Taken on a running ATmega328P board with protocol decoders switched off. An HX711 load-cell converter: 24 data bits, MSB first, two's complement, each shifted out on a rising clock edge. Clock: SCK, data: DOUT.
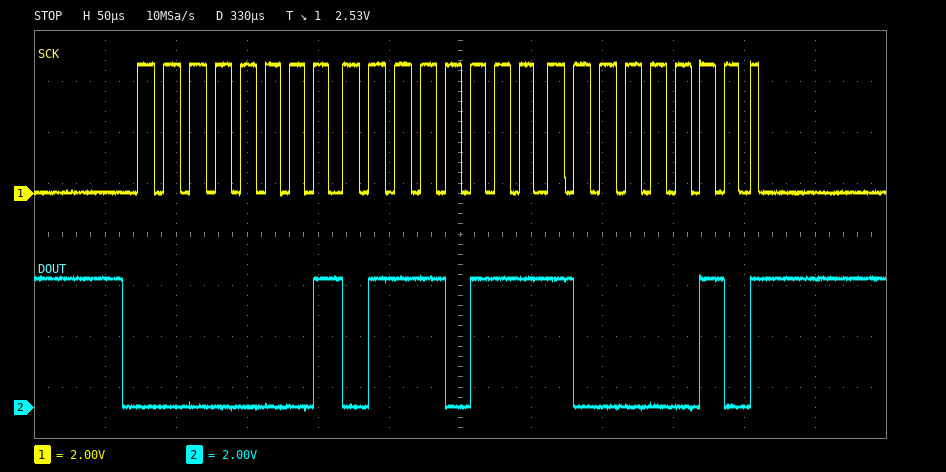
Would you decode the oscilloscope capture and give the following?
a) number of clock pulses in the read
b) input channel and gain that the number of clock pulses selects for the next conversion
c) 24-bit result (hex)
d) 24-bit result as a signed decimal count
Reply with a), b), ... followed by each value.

a) 25
b) channel A, gain 128
c) 0x017782
d) 96130
